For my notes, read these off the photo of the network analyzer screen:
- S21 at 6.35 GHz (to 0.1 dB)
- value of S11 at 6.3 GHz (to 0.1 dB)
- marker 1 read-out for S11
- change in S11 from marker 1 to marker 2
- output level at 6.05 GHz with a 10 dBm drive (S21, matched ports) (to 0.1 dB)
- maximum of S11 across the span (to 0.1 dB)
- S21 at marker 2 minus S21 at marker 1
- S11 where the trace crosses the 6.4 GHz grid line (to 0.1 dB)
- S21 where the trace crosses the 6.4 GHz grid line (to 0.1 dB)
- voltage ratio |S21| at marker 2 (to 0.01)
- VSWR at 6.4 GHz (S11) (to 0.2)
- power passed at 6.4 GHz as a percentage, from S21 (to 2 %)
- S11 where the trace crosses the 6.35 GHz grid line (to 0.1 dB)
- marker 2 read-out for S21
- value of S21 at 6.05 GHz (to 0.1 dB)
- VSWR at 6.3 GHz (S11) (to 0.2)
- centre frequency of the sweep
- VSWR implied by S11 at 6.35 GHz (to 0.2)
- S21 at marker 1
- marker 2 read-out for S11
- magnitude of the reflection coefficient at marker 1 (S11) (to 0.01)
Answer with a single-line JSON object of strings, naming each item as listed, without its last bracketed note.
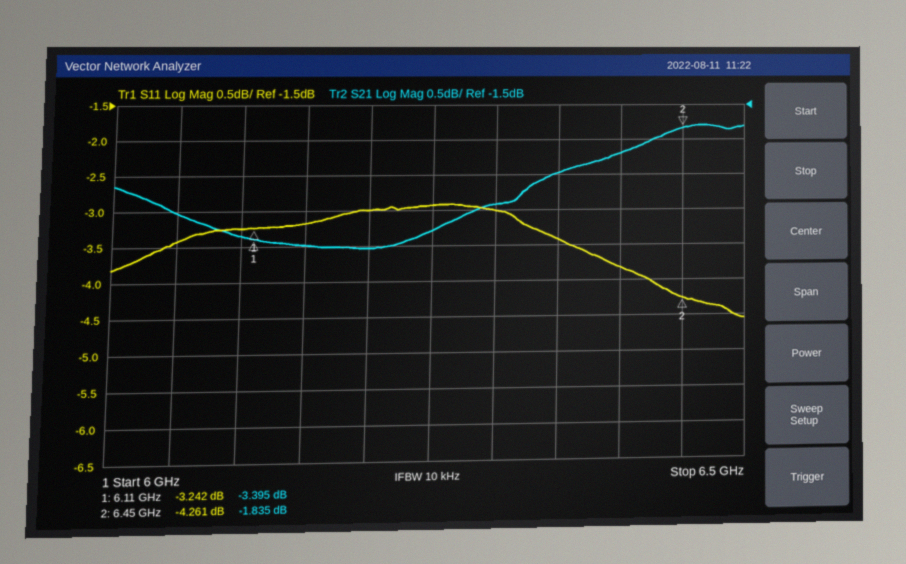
{"S21 at 6.35 GHz": "-2.5 dB", "value of S11 at 6.3 GHz": "-3.0 dB", "marker 1 read-out for S11": "-3.242 dB", "change in S11 from marker 1 to marker 2": "-1.019 dB", "output level at 6.05 GHz with a 10 dBm drive (S21, matched ports)": "7.0 dBm", "maximum of S11 across the span": "-2.9 dB", "S21 at marker 2 minus S21 at marker 1": "1.560 dB", "S11 where the trace crosses the 6.4 GHz grid line": "-3.8 dB", "S21 where the trace crosses the 6.4 GHz grid line": "-2.2 dB", "voltage ratio |S21| at marker 2": "0.81", "VSWR at 6.4 GHz (S11)": "4.6", "power passed at 6.4 GHz as a percentage, from S21": "60 %", "S11 where the trace crosses the 6.35 GHz grid line": "-3.4 dB", "marker 2 read-out for S21": "-1.835 dB", "value of S21 at 6.05 GHz": "-3.0 dB", "VSWR at 6.3 GHz (S11)": "5.8", "centre frequency of the sweep": "6.25 GHz", "VSWR implied by S11 at 6.35 GHz": "5.2", "S21 at marker 1": "-3.395 dB", "marker 2 read-out for S11": "-4.261 dB", "magnitude of the reflection coefficient at marker 1 (S11)": "0.69"}
